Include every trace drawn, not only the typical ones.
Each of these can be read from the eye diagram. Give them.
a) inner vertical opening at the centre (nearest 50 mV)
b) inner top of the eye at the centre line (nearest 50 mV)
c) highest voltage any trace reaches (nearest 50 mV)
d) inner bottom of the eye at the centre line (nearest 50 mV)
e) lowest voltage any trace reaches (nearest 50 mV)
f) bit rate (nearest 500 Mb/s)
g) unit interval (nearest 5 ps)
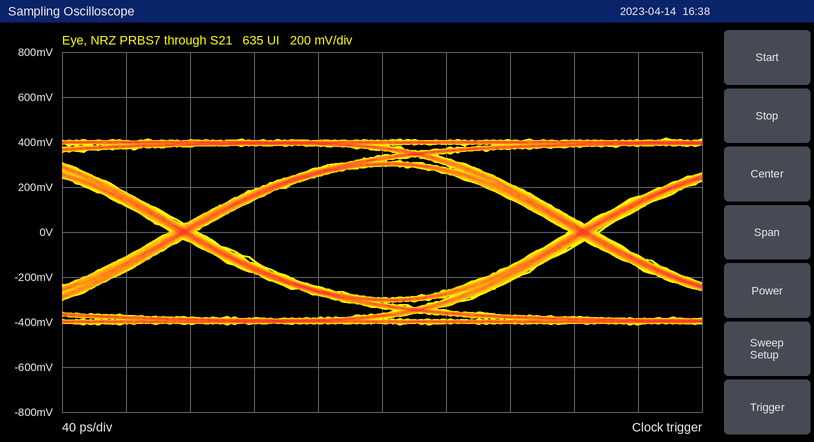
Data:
600 mV
300 mV
400 mV
-300 mV
-400 mV
4.0 Gb/s
250 ps
